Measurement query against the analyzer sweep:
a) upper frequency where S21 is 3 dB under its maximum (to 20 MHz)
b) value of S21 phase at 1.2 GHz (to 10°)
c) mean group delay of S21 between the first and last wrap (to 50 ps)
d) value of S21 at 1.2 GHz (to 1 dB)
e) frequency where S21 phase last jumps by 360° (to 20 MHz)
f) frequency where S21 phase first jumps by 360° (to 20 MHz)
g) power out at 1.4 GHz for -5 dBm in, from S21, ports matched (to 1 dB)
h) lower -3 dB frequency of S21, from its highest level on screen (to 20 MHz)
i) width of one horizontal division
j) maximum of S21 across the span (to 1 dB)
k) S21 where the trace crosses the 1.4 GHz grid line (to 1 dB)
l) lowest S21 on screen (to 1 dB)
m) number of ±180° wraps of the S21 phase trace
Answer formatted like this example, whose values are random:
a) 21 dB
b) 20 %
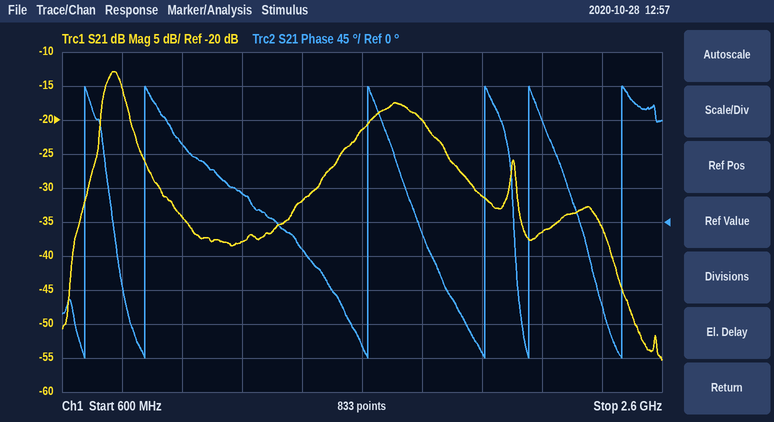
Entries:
a) 800 MHz
b) 40°
c) 2.80 ns
d) -38 dB
e) 2.46 GHz
f) 680 MHz
g) -37 dBm
h) 740 MHz
i) 200 MHz
j) -13 dB
k) -32 dB
l) -55 dB
m) 6
